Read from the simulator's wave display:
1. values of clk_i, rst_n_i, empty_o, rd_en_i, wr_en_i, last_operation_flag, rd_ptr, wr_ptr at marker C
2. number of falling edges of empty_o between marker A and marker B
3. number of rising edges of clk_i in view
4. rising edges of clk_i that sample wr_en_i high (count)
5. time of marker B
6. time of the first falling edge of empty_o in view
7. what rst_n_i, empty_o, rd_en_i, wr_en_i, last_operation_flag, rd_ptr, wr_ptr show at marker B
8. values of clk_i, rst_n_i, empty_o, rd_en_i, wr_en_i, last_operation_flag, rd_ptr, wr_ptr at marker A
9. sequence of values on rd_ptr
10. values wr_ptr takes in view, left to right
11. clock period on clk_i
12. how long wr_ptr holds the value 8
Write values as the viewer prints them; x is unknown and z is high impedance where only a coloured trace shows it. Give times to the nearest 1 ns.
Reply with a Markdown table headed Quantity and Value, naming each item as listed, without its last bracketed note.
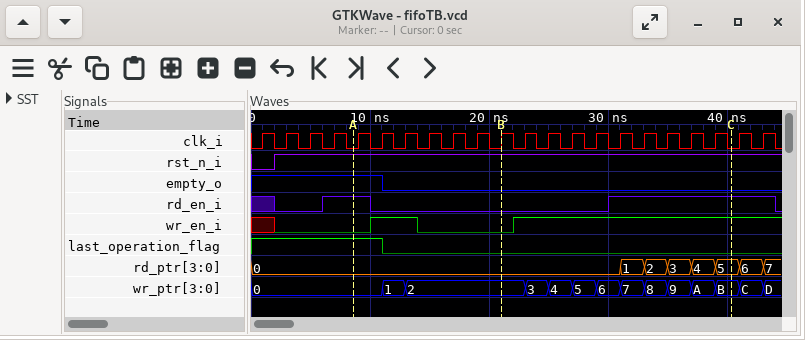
| Quantity | Value |
|---|---|
| values of clk_i, rst_n_i, empty_o, rd_en_i, wr_en_i, last_operation_flag, rd_ptr, wr_ptr at marker C | clk_i=0, rst_n_i=1, empty_o=0, rd_en_i=1, wr_en_i=1, last_operation_flag=0, rd_ptr=5, wr_ptr=B |
| number of falling edges of empty_o between marker A and marker B | 1 |
| number of rising edges of clk_i in view | 22 |
| rising edges of clk_i that sample wr_en_i high | 13 |
| time of marker B | 21 ns |
| time of the first falling edge of empty_o in view | 11 ns |
| what rst_n_i, empty_o, rd_en_i, wr_en_i, last_operation_flag, rd_ptr, wr_ptr show at marker B | rst_n_i=1, empty_o=0, rd_en_i=0, wr_en_i=0, last_operation_flag=0, rd_ptr=0, wr_ptr=2 |
| values of clk_i, rst_n_i, empty_o, rd_en_i, wr_en_i, last_operation_flag, rd_ptr, wr_ptr at marker A | clk_i=0, rst_n_i=1, empty_o=1, rd_en_i=1, wr_en_i=0, last_operation_flag=1, rd_ptr=0, wr_ptr=0 |
| sequence of values on rd_ptr | 0, 1, 2, 3, 4, 5, 6, 7 |
| values wr_ptr takes in view, left to right | 0, 1, 2, 3, 4, 5, 6, 7, 8, 9, A, B, C, D |
| clock period on clk_i | 2 ns |
| how long wr_ptr holds the value 8 | 2 ns |
